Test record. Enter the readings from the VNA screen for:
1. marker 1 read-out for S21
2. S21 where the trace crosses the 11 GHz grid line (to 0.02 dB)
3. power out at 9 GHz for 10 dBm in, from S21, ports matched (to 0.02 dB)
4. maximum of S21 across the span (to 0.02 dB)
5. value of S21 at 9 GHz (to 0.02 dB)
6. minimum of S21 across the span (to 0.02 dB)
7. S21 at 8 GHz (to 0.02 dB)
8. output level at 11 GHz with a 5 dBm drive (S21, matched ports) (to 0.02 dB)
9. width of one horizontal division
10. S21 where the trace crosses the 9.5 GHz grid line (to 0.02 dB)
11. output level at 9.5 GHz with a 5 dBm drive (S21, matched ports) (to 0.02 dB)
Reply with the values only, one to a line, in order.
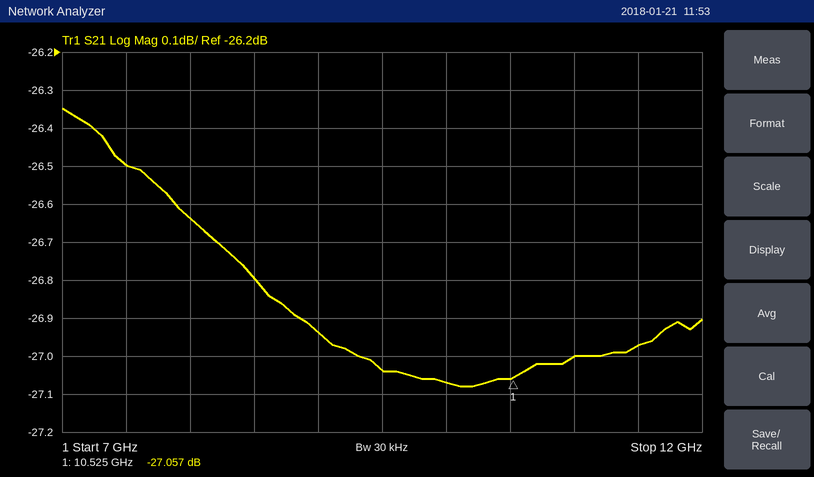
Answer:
-27.057 dB
-27.00 dB
-16.94 dBm
-26.34 dB
-26.94 dB
-27.08 dB
-26.64 dB
-22.00 dBm
500 MHz
-27.04 dB
-22.04 dBm
